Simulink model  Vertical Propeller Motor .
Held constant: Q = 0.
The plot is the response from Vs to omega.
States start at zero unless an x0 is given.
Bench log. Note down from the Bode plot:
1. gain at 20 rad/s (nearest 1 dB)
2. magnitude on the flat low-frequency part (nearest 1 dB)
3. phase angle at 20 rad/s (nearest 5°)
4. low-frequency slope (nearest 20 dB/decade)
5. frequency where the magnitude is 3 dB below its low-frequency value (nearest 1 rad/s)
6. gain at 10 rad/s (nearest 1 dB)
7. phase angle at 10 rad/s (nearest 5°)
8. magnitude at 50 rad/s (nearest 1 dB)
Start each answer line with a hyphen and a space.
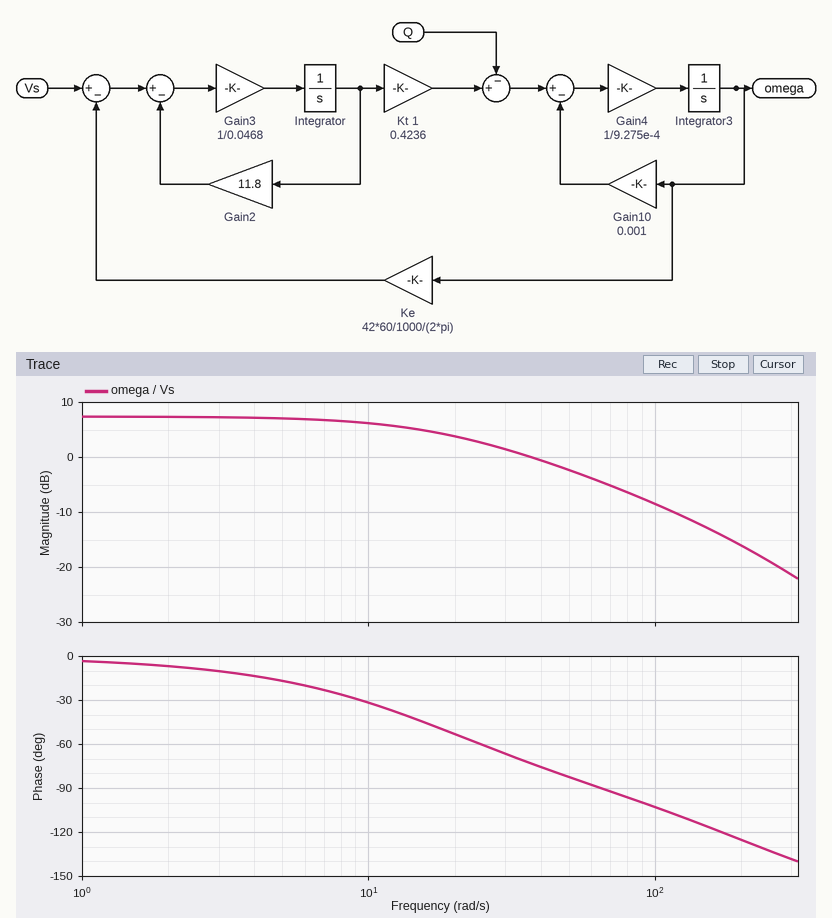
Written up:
- 4 dB
- 7 dB
- -55°
- 0 dB/decade
- 18 rad/s
- 6 dB
- -30°
- -2 dB
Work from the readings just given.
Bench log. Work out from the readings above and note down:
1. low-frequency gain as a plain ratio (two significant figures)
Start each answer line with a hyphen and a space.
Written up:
- 2.2
